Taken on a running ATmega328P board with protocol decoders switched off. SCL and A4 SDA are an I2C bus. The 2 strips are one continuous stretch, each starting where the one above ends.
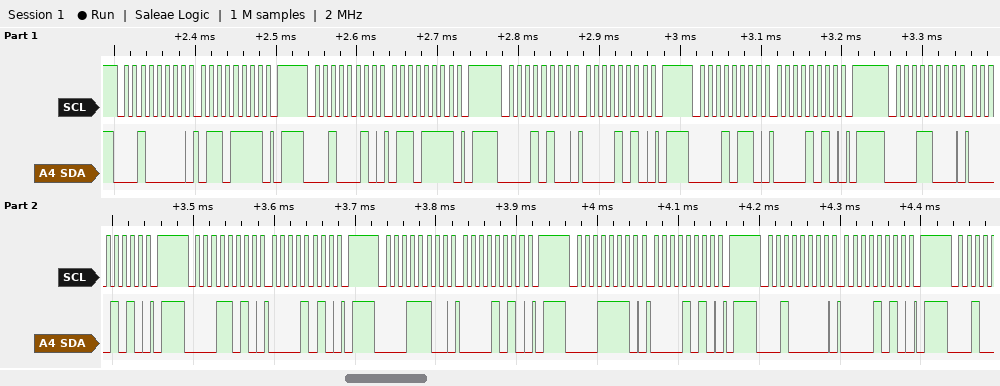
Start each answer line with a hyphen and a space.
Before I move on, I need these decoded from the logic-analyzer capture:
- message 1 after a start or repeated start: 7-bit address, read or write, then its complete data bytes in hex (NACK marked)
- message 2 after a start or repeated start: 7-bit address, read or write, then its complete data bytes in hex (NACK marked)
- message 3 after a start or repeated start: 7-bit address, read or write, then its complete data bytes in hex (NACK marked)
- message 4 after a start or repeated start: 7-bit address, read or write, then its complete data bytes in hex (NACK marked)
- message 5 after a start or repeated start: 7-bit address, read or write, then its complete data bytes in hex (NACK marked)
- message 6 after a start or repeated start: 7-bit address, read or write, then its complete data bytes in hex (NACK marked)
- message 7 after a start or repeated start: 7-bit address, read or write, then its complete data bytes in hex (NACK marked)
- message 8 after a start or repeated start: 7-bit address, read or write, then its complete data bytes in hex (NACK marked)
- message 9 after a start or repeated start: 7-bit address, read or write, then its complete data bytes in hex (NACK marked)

- 0x10 write: 6F
- 0x11 write: 6F
- 0x0A write: 0A
- 0x0B write: 0A
- 0x0C write: 0A
- 0x0D write: 0A
- 0x0E write: 0A
- 0x0F write: 0A
- 0x10 write: 0A
